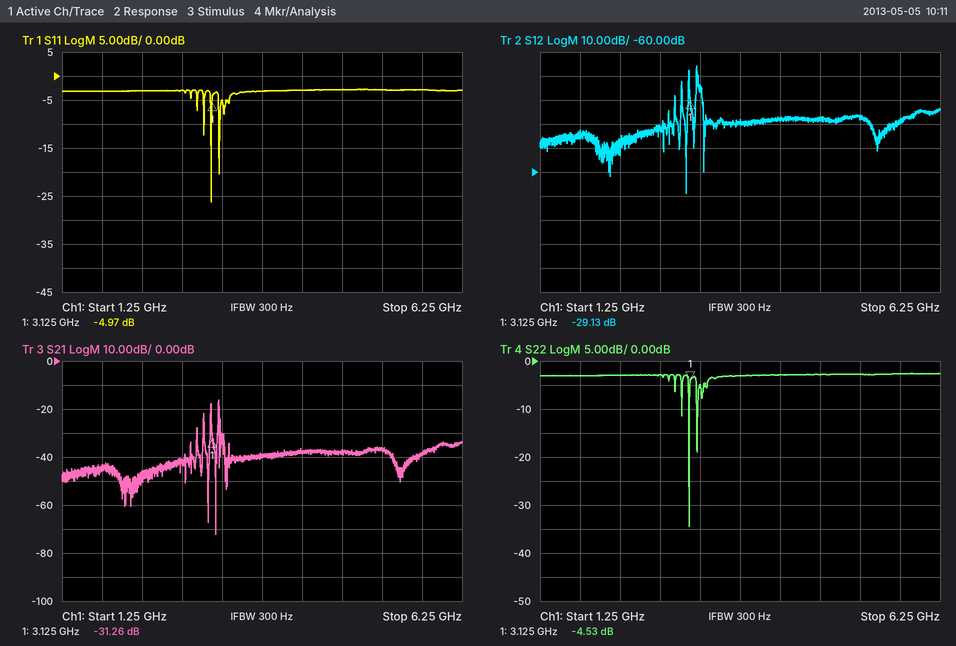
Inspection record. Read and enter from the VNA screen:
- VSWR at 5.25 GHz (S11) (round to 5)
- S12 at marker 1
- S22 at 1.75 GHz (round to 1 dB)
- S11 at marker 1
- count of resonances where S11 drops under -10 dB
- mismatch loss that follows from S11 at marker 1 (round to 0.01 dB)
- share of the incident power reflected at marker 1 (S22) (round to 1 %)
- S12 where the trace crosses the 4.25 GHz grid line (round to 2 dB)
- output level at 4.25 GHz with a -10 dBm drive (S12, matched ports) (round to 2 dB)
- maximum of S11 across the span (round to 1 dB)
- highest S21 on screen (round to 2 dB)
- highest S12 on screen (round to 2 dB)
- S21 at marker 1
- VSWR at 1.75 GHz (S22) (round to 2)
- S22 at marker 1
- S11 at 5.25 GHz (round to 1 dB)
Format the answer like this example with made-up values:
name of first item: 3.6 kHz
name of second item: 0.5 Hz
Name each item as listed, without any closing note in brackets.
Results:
VSWR at 5.25 GHz (S11): 5
S12 at marker 1: -29.13 dB
S22 at 1.75 GHz: -3 dB
S11 at marker 1: -4.97 dB
count of resonances where S11 drops under -10 dB: 3
mismatch loss that follows from S11 at marker 1: 1.66 dB
share of the incident power reflected at marker 1 (S22): 35 %
S12 where the trace crosses the 4.25 GHz grid line: -38 dB
output level at 4.25 GHz with a -10 dBm drive (S12, matched ports): -48 dBm
maximum of S11 across the span: -3 dB
highest S21 on screen: -16 dB
highest S12 on screen: -16 dB
S21 at marker 1: -31.26 dB
VSWR at 1.75 GHz (S22): 6
S22 at marker 1: -4.53 dB
S11 at 5.25 GHz: -3 dB
